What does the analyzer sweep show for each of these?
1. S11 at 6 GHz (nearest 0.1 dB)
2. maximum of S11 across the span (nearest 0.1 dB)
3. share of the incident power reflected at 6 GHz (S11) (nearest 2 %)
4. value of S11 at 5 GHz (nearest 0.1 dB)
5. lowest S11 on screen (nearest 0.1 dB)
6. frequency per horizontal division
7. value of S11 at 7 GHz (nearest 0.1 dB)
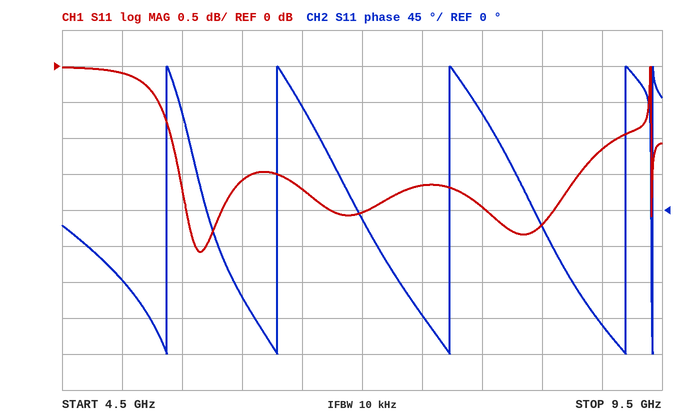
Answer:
-1.6 dB
0.0 dB
70 %
-0.1 dB
-2.6 dB
500 MHz
-2.0 dB
